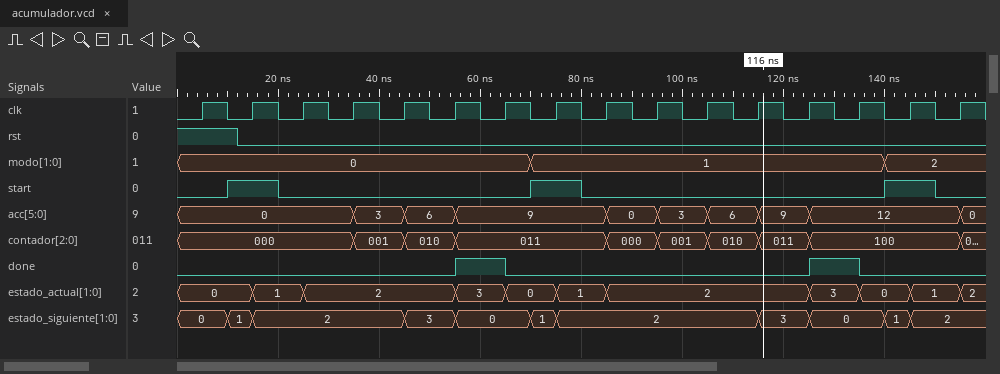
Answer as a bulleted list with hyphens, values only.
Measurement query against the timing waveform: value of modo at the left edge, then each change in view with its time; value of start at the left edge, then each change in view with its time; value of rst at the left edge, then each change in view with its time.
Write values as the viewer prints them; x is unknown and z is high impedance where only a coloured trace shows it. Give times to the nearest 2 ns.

- 0, 1 at 70 ns, 2 at 140 ns
- 0, 1 at 10 ns, 0 at 20 ns, 1 at 70 ns, 0 at 80 ns, 1 at 140 ns, 0 at 150 ns
- 1, 0 at 12 ns
